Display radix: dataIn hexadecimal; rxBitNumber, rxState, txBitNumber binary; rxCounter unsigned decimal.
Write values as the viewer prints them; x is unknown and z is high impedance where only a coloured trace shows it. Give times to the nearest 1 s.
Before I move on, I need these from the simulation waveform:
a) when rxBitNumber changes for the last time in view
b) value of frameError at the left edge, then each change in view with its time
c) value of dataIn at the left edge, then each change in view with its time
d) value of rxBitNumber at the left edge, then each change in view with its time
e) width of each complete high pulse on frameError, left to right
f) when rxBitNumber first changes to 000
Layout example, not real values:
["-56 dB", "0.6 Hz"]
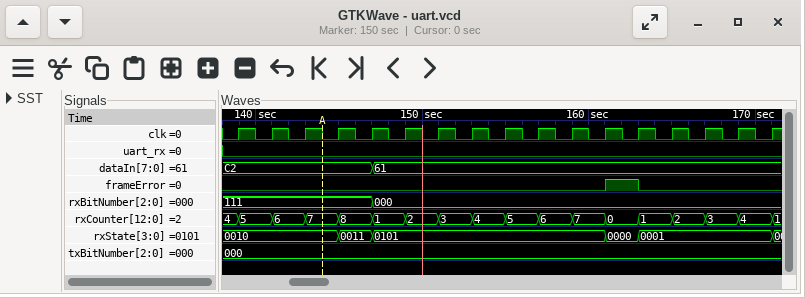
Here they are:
["147 s", "0, 1 at 161 s, 0 at 163 s", "C2, 61 at 147 s", "111, 000 at 147 s", "2 s", "147 s"]
